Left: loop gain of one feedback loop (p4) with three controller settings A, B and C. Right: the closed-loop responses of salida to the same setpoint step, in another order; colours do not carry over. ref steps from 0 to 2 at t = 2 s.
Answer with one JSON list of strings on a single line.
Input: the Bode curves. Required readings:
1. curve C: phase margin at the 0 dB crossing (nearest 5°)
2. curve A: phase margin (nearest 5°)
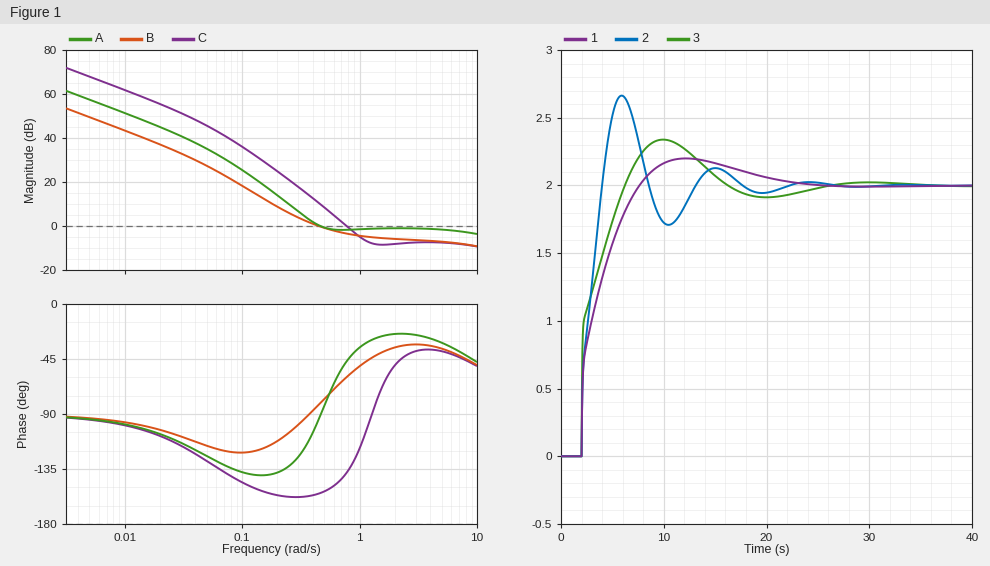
["40°", "90°"]
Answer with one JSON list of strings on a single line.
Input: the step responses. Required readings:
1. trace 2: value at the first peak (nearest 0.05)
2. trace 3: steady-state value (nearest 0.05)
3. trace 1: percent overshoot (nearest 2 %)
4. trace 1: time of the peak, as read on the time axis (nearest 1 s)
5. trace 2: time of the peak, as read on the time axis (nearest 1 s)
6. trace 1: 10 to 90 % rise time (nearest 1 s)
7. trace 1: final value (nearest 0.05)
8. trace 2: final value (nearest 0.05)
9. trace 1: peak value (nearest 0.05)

["2.65", "2.00", "10 %", "12 s", "6 s", "4 s", "2.00", "2.00", "2.20"]
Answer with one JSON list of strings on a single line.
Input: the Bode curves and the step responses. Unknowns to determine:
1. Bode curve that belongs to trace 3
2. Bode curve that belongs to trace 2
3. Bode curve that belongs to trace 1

["A", "C", "B"]
